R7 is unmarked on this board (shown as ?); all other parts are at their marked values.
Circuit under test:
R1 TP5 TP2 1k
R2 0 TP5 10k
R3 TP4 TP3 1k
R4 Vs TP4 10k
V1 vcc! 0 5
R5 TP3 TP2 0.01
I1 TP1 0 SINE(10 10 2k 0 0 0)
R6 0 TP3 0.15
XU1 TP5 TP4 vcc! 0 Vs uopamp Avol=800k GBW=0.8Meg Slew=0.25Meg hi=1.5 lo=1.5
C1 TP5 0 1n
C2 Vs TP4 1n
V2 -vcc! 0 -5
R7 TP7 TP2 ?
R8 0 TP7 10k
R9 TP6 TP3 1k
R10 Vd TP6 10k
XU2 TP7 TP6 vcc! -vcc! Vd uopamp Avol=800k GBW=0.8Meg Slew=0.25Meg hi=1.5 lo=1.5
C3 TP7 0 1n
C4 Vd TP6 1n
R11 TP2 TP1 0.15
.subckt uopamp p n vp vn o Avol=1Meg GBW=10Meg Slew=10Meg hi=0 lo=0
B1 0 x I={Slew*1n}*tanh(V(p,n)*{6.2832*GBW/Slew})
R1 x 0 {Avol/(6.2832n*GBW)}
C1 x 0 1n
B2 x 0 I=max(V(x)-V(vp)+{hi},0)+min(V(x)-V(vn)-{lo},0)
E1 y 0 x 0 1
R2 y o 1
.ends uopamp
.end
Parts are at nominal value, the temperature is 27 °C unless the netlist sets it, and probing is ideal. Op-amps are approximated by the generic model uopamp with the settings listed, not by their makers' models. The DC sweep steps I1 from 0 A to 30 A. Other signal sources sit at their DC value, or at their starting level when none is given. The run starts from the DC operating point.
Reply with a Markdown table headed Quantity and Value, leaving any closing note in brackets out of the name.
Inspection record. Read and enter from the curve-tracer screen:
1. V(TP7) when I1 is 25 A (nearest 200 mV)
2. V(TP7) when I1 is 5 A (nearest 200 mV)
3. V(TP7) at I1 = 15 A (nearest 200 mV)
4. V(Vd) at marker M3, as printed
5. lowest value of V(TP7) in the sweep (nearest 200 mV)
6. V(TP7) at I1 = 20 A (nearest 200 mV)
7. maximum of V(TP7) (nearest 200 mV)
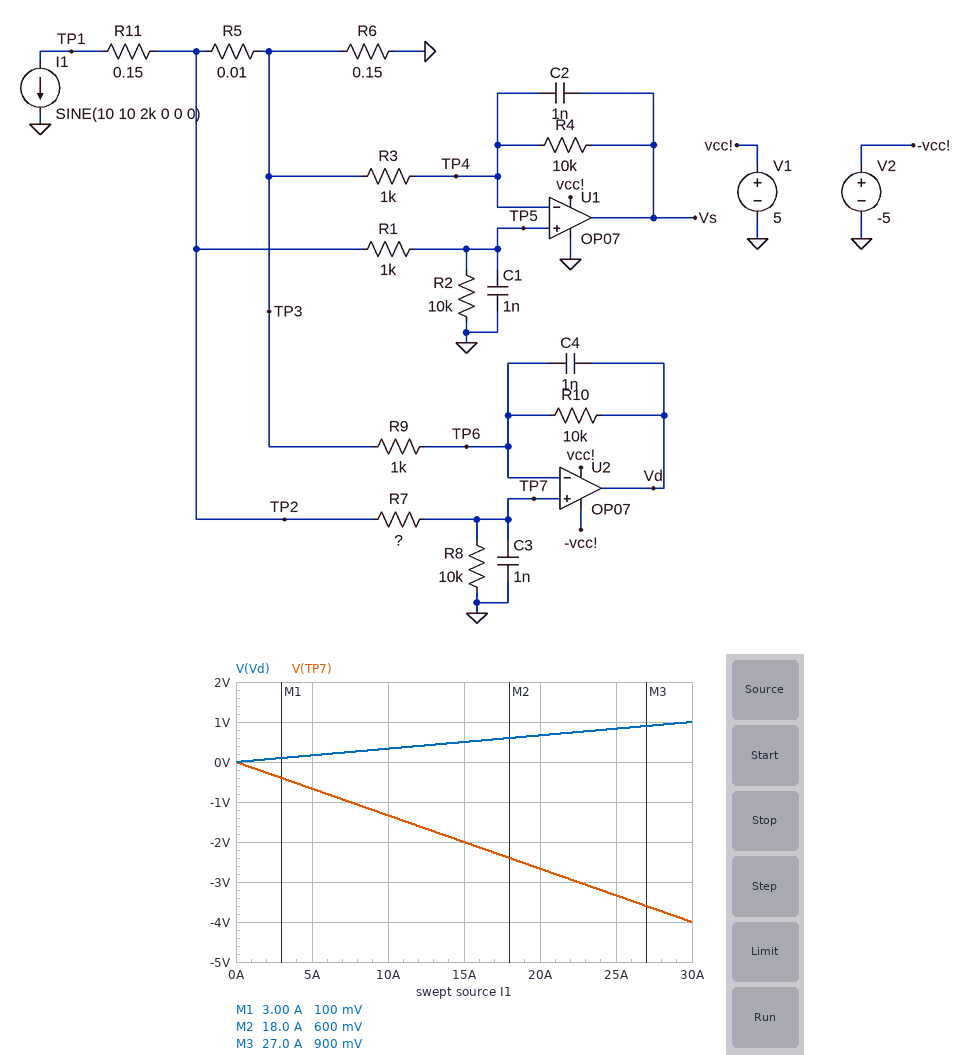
| Quantity | Value |
|---|---|
| V(TP7) when I1 is 25 A | -3.4 V |
| V(TP7) when I1 is 5 A | -600 mV |
| V(TP7) at I1 = 15 A | -2.0 V |
| V(Vd) at marker M3, as printed | 900 mV |
| lowest value of V(TP7) in the sweep | -4.0 V |
| V(TP7) at I1 = 20 A | -2.6 V |
| maximum of V(TP7) | 0 V |
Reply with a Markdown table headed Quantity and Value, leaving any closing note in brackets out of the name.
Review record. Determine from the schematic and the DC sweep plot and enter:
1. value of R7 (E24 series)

| Quantity | Value |
|---|---|
| value of R7 | 2 kΩ |
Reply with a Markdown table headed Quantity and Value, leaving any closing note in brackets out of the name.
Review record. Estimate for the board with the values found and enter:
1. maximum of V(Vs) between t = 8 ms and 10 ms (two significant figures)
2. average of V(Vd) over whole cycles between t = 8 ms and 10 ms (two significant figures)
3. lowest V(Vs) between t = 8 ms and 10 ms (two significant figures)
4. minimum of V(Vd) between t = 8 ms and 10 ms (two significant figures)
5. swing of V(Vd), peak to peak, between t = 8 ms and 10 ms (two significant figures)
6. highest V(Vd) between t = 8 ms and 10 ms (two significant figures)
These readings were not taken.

| Quantity | Value |
|---|---|
| maximum of V(Vs) between t = 8 ms and 10 ms | 1.5 V |
| average of V(Vd) over whole cycles between t = 8 ms and 10 ms | 330 mV |
| lowest V(Vs) between t = 8 ms and 10 ms | 1.5 V |
| minimum of V(Vd) between t = 8 ms and 10 ms | -27 mV |
| swing of V(Vd), peak to peak, between t = 8 ms and 10 ms | 720 mV |
| highest V(Vd) between t = 8 ms and 10 ms | 690 mV |
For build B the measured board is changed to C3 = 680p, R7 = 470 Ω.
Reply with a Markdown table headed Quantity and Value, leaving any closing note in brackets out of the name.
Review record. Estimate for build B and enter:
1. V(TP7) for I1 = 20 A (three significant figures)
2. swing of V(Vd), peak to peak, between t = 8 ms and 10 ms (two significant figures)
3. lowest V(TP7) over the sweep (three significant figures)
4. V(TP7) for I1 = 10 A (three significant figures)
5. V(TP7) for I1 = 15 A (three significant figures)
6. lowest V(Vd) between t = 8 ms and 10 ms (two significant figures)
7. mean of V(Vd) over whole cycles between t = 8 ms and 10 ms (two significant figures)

| Quantity | Value |
|---|---|
| V(TP7) for I1 = 20 A | -3.06 V |
| swing of V(Vd), peak to peak, between t = 8 ms and 10 ms | 3.5 V |
| lowest V(TP7) over the sweep | -4.58 V |
| V(TP7) for I1 = 10 A | -1.53 V |
| V(TP7) for I1 = 15 A | -2.29 V |
| lowest V(Vd) between t = 8 ms and 10 ms | -3.5 V |
| mean of V(Vd) over whole cycles between t = 8 ms and 10 ms | -1.8 V |
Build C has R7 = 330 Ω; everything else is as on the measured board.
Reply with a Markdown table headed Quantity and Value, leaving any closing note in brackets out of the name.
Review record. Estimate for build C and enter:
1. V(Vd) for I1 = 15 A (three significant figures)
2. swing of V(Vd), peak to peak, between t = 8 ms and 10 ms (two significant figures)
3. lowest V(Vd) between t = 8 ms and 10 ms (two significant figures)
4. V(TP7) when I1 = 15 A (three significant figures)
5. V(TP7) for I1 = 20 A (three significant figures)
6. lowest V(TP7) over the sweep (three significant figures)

| Quantity | Value |
|---|---|
| V(Vd) for I1 = 15 A | -3.06 V |
| swing of V(Vd), peak to peak, between t = 8 ms and 10 ms | 3.5 V |
| lowest V(Vd) between t = 8 ms and 10 ms | -3.5 V |
| V(TP7) when I1 = 15 A | -2.32 V |
| V(TP7) for I1 = 20 A | -3.10 V |
| lowest V(TP7) over the sweep | -4.65 V |
